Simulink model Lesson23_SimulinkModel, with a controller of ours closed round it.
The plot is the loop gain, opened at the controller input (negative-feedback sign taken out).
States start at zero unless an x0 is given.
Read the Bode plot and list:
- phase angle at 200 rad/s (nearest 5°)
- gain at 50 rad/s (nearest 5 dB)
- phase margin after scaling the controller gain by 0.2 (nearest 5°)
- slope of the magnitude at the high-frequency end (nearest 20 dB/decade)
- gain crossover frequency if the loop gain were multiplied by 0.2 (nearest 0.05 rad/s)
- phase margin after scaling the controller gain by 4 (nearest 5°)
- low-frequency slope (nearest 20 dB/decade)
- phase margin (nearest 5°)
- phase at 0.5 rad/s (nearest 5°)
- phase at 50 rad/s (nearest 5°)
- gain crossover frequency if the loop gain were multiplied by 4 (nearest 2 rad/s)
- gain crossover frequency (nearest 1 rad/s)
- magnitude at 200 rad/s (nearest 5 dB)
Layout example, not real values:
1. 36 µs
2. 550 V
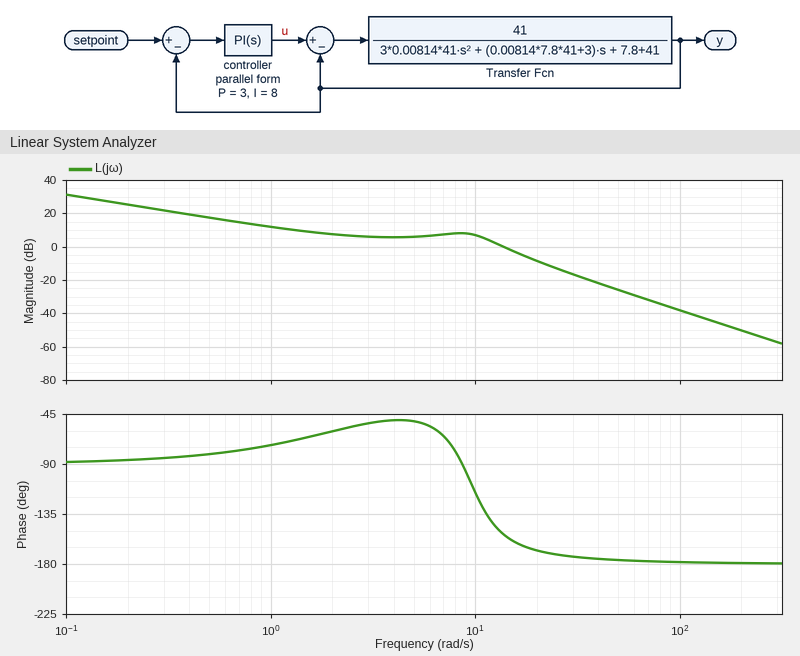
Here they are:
1. -180°
2. -25 dB
3. 105°
4. -40 dB/decade
5. 0.75 rad/s
6. 10°
7. -20 dB/decade
8. 25°
9. -80°
10. -175°
11. 24 rad/s
12. 14 rad/s
13. -50 dB
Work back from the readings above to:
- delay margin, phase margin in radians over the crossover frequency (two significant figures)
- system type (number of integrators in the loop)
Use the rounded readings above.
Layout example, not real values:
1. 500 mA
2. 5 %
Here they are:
1. 0.031 s
2. 1
